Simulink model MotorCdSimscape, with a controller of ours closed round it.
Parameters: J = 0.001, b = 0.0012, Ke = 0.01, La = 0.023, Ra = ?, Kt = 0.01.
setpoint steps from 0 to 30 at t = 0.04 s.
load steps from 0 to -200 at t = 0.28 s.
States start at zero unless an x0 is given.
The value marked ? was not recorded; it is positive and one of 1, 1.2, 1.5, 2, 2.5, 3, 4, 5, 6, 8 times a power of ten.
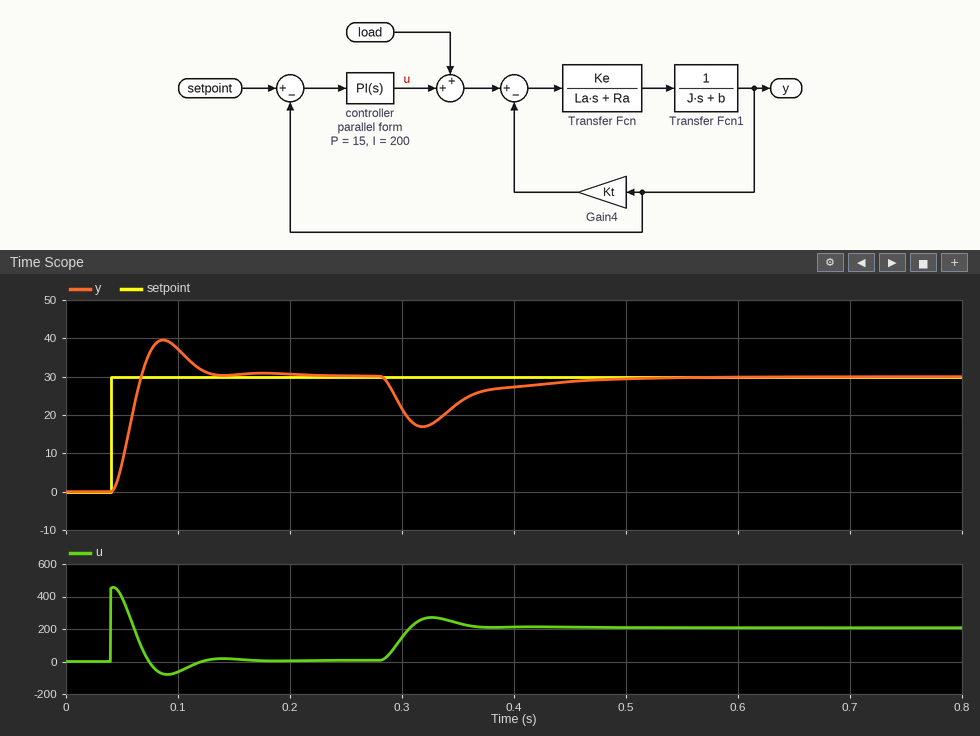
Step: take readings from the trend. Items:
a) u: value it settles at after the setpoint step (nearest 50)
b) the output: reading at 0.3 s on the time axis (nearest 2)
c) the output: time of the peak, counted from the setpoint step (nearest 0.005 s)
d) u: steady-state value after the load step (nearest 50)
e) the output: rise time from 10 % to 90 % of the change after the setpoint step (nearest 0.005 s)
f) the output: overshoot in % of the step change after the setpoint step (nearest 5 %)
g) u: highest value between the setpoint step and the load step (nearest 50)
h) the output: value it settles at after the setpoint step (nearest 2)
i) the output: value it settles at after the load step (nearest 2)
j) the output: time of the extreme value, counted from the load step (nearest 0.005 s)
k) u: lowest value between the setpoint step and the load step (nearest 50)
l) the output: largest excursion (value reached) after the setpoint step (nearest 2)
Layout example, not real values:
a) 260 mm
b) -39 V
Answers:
a) 0
b) 22
c) 0.045 s
d) 200
e) 0.020 s
f) 30 %
g) 450
h) 30
i) 30
j) 0.040 s
k) -100
l) 40
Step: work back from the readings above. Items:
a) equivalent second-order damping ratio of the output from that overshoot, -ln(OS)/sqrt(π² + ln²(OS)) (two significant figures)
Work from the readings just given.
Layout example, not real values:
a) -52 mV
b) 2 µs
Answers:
a) 0.36
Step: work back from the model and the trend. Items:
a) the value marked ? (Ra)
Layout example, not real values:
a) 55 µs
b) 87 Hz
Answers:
a) 2
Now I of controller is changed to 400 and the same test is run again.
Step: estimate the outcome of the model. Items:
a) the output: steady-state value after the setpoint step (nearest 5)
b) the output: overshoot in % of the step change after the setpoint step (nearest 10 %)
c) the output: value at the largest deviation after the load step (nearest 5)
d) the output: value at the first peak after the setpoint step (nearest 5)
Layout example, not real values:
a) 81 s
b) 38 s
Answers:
a) 30
b) 50 %
c) 20
d) 45
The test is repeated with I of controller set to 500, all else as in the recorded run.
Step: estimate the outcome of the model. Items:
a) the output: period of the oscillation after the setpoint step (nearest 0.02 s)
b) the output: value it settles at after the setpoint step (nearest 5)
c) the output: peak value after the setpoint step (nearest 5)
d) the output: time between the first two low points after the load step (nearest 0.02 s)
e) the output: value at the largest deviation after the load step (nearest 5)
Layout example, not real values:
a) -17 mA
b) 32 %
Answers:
a) 0.10 s
b) 30
c) 45
d) 0.10 s
e) 20
